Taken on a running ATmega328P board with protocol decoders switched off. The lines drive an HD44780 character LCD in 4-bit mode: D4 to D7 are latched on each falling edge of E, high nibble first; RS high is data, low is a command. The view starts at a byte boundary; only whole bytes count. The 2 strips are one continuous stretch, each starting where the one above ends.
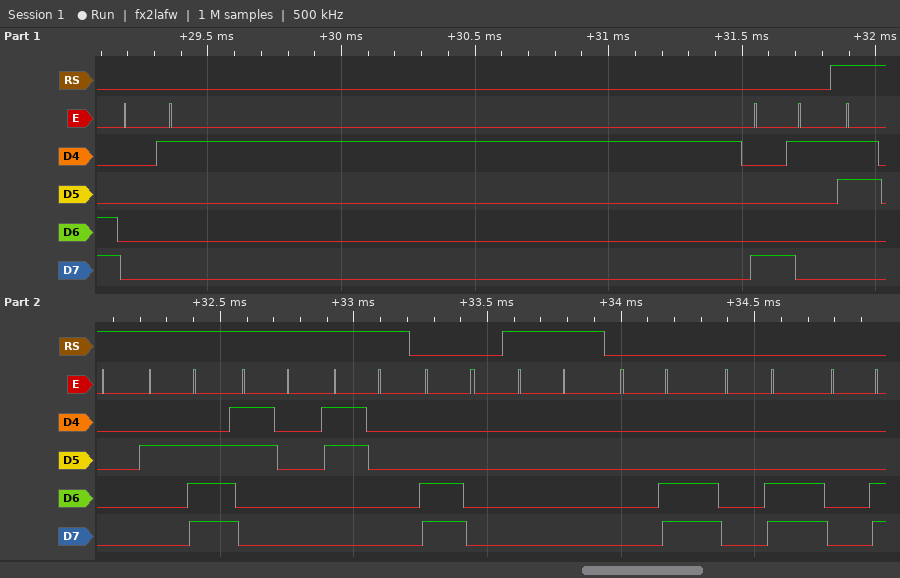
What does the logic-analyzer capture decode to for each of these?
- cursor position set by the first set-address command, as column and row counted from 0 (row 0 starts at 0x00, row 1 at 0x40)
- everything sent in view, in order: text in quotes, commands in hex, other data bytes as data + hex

column 1, row 0
0x01 0x81 "0.00" 0xC0 data 00 0x0C 0x0C 0x0C
